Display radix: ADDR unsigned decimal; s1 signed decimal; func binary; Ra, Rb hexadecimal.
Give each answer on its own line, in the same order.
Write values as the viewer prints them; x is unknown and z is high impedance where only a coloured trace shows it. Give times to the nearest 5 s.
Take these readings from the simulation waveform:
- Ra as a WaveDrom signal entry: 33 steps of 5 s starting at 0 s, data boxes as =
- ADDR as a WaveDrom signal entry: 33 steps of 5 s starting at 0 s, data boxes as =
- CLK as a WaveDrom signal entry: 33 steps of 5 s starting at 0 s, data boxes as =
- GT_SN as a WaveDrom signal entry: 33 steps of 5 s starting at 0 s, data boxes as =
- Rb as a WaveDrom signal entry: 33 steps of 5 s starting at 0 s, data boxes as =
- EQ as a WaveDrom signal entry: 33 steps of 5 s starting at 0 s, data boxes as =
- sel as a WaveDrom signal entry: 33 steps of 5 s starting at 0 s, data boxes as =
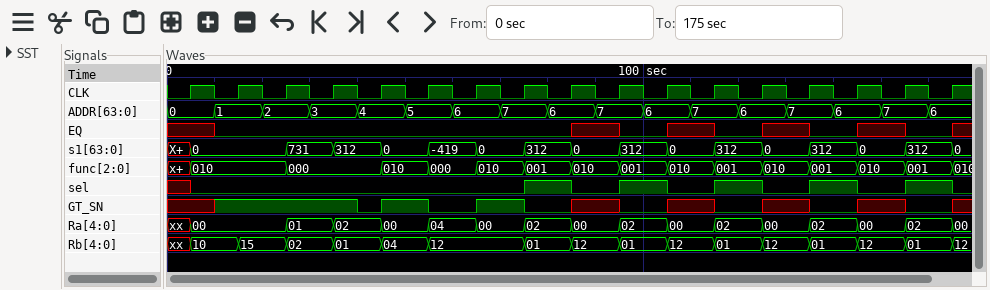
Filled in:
{name: 'Ra', wave: 'x=...=.=.=.=.=.=.=.=.=.=.=.=.=.=.', data: '00 01 02 00 04 00 02 00 02 00 02 00 02 00 02'}
{name: 'ADDR', wave: '=.=.=.=.=.=.=.=.=.=.=.=.=.=.=.=.=', data: '0 1 2 3 4 5 6 7 6 7 6 7 6 7 6 7 6'}
{name: 'CLK', wave: '010101010101010101010101010101010'}
{name: 'GT_SN', wave: 'x.1.....01.0.1.0.x.0.x.0.x.0.x.0.'}
{name: 'Rb', wave: 'x=.=.=.=.=.=...=.=.=.=.=.=.=.=.=.', data: '10 15 02 01 04 12 01 12 01 12 01 12 01 12 01'}
{name: 'EQ', wave: 'x.0..............x.0.x.0.x.0.x.0.'}
{name: 'sel', wave: 'x0.............1.0.1.0.1.0.1.0.1.'}
